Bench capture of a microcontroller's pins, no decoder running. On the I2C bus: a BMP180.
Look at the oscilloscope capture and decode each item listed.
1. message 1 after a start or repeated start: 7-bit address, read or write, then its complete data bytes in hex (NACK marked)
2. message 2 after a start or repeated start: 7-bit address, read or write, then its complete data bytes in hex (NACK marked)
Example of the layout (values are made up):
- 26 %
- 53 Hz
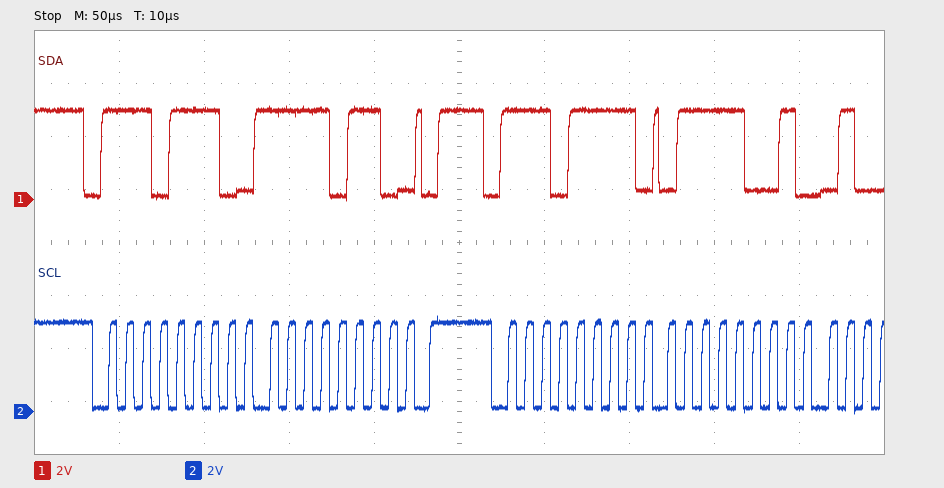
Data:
- 0x77 write: F6
- 0x77 read: 79
